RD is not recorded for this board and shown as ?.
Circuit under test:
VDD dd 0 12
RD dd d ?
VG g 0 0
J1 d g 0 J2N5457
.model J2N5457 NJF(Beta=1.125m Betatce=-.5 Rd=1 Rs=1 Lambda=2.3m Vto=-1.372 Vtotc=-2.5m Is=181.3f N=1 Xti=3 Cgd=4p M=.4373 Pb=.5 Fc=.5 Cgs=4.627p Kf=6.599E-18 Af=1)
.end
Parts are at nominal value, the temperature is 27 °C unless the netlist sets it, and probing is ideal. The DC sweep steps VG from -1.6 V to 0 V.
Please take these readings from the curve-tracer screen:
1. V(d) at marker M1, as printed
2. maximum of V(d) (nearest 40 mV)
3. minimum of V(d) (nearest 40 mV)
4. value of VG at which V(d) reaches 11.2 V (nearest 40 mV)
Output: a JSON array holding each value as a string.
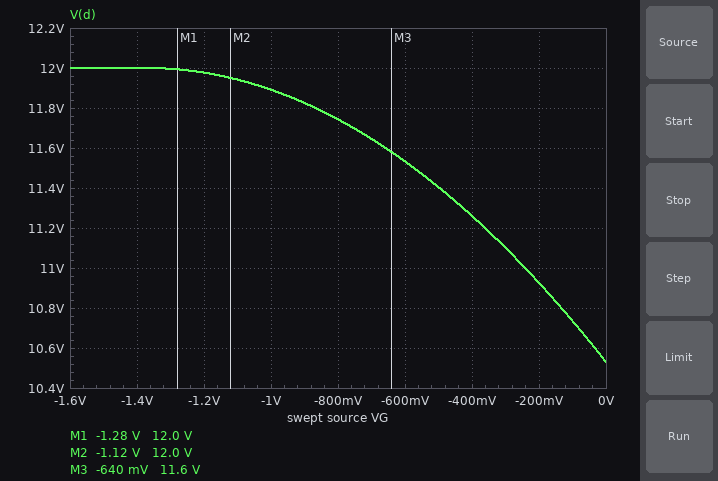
["12.0 V", "12.00 V", "10.52 V", "-360 mV"]
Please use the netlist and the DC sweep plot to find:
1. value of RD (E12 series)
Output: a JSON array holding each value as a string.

["680 Ω"]
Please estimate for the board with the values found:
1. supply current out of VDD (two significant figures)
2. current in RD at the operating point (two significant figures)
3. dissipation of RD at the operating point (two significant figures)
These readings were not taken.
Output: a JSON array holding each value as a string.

["2.2 mA", "2.2 mA", "3.2 mW"]
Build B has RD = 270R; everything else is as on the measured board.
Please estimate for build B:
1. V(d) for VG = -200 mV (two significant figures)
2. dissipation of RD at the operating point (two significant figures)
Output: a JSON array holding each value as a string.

["12 V", "1.3 mW"]
